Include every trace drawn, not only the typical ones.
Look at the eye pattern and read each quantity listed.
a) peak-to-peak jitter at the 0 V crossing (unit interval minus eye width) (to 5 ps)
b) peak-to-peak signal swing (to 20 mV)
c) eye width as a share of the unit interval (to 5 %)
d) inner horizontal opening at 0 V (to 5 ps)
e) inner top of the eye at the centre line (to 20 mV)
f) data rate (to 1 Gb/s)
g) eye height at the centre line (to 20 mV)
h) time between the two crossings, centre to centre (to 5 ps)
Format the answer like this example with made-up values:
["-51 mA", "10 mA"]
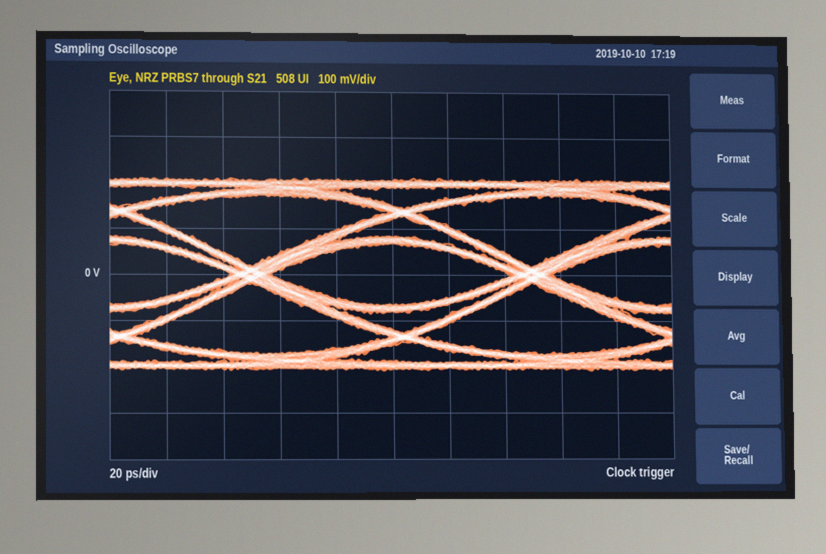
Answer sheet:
["15 ps", "420 mV", "85 %", "85 ps", "60 mV", "10 Gb/s", "140 mV", "100 ps"]
